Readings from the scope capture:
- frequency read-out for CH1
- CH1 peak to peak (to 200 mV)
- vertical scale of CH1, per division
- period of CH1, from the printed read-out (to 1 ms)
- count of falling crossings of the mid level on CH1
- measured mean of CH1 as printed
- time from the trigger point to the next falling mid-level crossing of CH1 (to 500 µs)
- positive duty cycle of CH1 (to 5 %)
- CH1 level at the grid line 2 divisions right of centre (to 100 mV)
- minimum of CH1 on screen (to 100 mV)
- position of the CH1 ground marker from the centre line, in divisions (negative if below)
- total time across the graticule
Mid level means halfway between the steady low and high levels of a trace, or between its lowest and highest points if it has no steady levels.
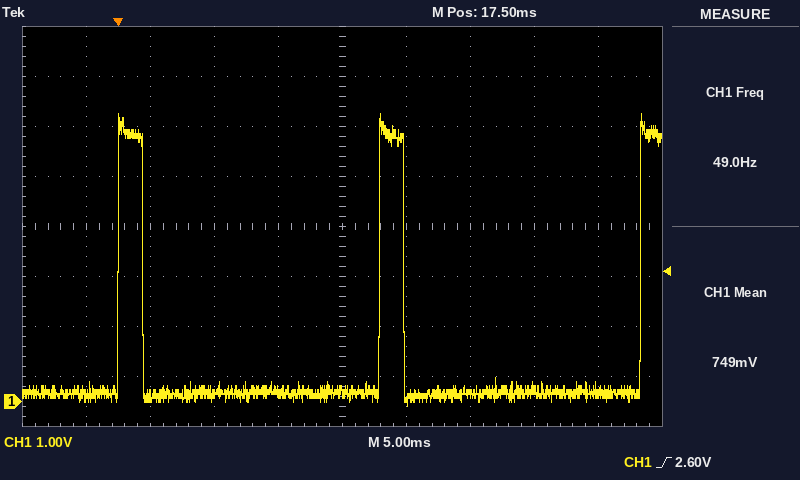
49.0 Hz
5.8 V
1 V
20 ms
2
749 mV
2.0 ms
10 %
200 mV
-100 mV
-3.5 div
50 ms
